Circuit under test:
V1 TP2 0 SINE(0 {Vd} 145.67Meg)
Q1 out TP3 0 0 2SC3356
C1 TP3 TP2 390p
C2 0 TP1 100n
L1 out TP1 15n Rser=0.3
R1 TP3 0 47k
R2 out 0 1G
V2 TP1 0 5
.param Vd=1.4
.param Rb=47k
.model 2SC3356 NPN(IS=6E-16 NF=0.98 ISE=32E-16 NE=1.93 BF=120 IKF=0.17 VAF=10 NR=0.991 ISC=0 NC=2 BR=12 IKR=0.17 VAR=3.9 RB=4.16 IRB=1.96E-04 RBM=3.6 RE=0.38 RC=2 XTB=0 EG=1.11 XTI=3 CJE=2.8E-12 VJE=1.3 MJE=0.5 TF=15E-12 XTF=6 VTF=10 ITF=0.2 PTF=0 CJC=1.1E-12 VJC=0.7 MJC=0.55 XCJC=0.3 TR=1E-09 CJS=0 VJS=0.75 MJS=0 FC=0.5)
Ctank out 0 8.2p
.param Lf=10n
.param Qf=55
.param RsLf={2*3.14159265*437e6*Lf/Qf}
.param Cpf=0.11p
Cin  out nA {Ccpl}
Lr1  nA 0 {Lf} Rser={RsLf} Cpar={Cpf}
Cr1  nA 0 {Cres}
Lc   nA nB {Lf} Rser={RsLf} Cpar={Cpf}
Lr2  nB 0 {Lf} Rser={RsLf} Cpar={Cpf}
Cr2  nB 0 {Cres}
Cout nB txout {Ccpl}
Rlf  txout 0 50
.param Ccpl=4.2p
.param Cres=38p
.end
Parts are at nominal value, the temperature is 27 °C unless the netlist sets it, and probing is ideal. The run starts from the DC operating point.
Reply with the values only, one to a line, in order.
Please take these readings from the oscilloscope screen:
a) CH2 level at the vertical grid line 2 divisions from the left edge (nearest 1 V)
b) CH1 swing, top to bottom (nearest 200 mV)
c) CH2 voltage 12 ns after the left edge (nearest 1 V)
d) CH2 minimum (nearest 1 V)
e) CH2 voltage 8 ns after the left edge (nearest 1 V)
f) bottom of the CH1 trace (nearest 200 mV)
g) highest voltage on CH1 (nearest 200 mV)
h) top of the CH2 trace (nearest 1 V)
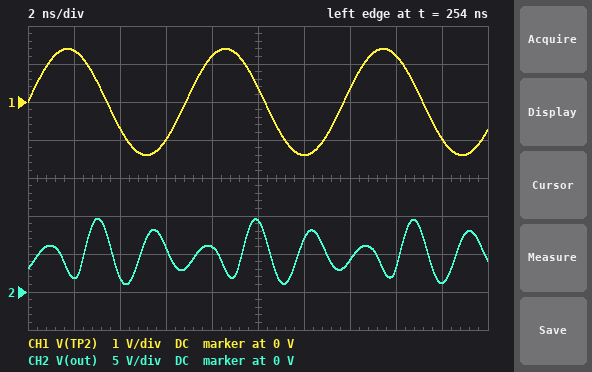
2 V
2.8 V
7 V
1 V
6 V
-1.4 V
1.4 V
10 V
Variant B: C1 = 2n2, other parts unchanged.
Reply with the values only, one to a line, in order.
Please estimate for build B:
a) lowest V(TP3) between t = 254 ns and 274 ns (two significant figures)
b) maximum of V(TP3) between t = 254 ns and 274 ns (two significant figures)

-1.8 V
1.0 V
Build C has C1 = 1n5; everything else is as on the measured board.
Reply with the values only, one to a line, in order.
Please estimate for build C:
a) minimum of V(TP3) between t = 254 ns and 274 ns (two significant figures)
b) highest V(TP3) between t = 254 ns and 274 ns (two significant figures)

-1.8 V
1.0 V
